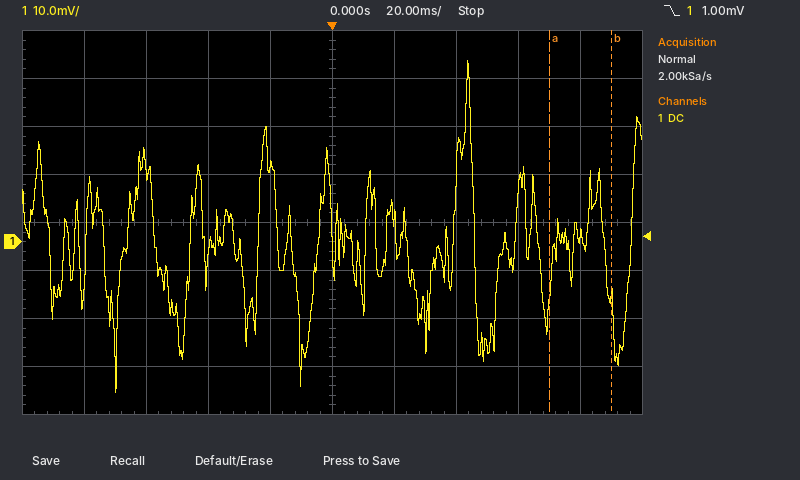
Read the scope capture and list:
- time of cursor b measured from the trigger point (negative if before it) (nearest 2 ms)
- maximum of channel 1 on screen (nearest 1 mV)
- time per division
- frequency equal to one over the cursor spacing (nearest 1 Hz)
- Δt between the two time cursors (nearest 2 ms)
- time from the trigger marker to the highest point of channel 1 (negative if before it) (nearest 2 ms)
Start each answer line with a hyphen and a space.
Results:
- +90 ms
- 38 mV
- 20 ms
- 50 Hz
- 20 ms
- +44 ms
